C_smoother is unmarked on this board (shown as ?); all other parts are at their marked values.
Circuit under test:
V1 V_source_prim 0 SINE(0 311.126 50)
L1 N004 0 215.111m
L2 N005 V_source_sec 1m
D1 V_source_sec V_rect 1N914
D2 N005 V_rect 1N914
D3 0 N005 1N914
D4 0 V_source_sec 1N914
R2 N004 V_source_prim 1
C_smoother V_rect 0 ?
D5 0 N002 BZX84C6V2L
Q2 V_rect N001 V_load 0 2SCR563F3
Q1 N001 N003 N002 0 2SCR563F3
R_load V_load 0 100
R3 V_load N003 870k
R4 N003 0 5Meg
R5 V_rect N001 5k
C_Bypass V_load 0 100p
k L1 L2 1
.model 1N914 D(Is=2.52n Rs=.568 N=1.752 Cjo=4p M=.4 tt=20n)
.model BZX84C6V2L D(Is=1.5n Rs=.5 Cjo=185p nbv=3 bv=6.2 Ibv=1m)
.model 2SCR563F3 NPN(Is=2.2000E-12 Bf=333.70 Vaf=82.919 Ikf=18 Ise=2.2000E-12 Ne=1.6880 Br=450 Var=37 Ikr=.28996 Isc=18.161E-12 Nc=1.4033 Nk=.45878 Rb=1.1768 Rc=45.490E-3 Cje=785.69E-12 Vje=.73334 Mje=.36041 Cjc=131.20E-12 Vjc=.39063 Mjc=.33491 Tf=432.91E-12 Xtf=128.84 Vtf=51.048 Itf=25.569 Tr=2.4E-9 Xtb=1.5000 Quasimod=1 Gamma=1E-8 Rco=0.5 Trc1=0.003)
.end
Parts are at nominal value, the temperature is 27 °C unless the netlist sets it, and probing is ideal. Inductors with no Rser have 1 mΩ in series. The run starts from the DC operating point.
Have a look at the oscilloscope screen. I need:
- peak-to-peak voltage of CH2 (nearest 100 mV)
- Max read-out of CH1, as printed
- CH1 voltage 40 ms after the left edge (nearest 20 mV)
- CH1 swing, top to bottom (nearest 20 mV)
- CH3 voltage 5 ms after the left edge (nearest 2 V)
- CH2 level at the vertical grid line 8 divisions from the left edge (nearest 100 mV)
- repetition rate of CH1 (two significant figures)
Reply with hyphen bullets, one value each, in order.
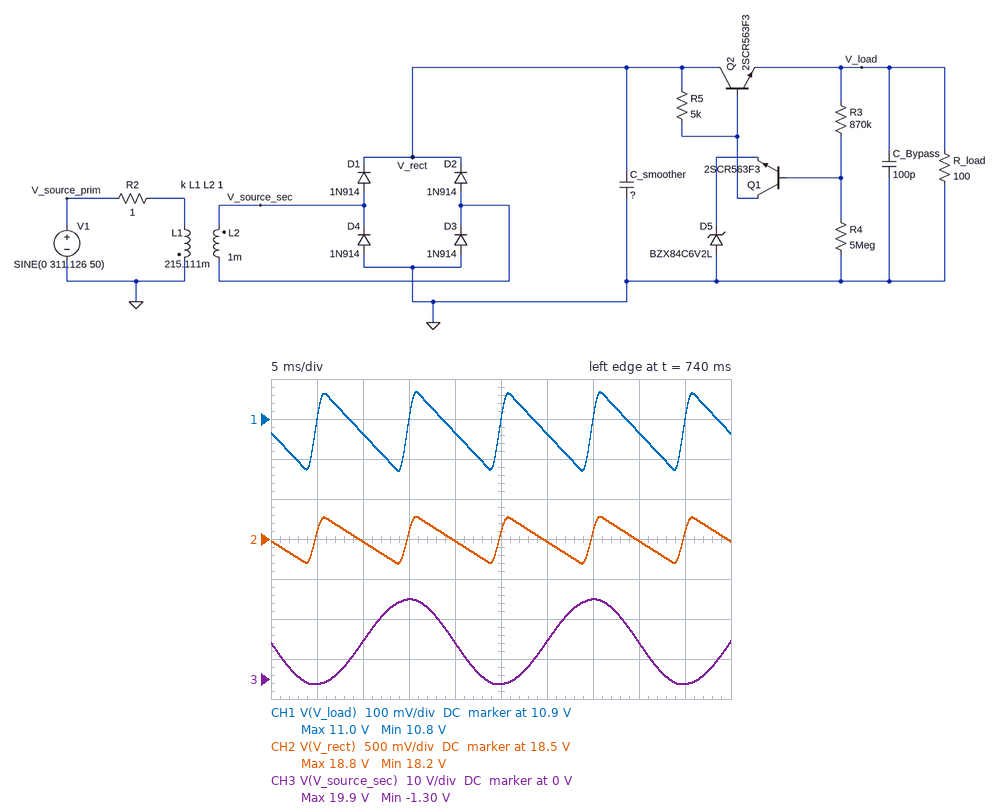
- 600 mV
- 11.0 V
- 10.86 V
- 200 mV
- -2 V
- 18.5 V
- 100 Hz
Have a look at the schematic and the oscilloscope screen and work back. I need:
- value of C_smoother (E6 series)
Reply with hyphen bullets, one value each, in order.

- 1.5 mF
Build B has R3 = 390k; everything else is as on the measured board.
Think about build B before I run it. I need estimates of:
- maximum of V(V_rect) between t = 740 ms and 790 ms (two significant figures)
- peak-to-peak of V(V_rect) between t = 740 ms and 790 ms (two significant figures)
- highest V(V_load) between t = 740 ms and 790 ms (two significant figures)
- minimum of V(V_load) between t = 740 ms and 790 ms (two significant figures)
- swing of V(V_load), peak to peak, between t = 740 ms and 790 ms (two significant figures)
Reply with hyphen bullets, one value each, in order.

- 19 V
- 500 mV
- 9.2 V
- 9.1 V
- 99 mV
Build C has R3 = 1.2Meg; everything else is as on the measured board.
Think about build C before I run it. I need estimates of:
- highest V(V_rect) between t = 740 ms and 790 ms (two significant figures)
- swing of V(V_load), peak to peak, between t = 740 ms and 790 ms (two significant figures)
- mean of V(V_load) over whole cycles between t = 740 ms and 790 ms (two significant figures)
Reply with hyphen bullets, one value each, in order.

- 19 V
- 250 mV
- 12 V
